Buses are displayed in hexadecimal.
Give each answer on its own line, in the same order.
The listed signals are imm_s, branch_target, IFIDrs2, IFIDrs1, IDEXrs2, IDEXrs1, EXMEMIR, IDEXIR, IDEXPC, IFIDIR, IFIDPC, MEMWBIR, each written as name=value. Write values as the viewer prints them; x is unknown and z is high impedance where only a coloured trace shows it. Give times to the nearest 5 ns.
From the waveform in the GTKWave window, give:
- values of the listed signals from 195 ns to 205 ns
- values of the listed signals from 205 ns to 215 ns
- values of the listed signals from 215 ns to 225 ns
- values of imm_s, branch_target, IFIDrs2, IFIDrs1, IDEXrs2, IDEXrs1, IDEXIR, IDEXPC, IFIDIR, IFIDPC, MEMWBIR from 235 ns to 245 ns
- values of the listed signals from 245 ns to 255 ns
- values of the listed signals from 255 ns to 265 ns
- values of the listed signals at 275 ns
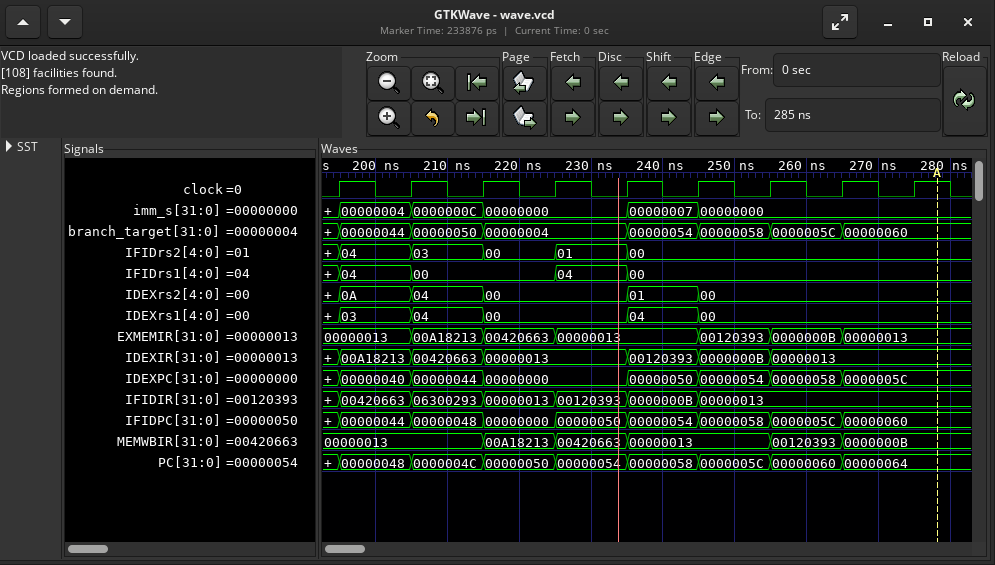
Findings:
imm_s=00000004, branch_target=00000044, IFIDrs2=04, IFIDrs1=04, IDEXrs2=0A, IDEXrs1=03, EXMEMIR=00000013, IDEXIR=00A18213, IDEXPC=00000040, IFIDIR=00420663, IFIDPC=00000044, MEMWBIR=00000013
imm_s=0000000C, branch_target=00000050, IFIDrs2=03, IFIDrs1=00, IDEXrs2=04, IDEXrs1=04, EXMEMIR=00A18213, IDEXIR=00420663, IDEXPC=00000044, IFIDIR=06300293, IFIDPC=00000048, MEMWBIR=00000013
imm_s=00000000, branch_target=00000004, IFIDrs2=00, IFIDrs1=00, IDEXrs2=00, IDEXrs1=00, EXMEMIR=00420663, IDEXIR=00000013, IDEXPC=00000000, IFIDIR=00000013, IFIDPC=00000000, MEMWBIR=00A18213
imm_s=00000007, branch_target=00000054, IFIDrs2=00, IFIDrs1=00, IDEXrs2=01, IDEXrs1=04, IDEXIR=00120393, IDEXPC=00000050, IFIDIR=0000000B, IFIDPC=00000054, MEMWBIR=00000013
imm_s=00000000, branch_target=00000058, IFIDrs2=00, IFIDrs1=00, IDEXrs2=00, IDEXrs1=00, EXMEMIR=00120393, IDEXIR=0000000B, IDEXPC=00000054, IFIDIR=00000013, IFIDPC=00000058, MEMWBIR=00000013
imm_s=00000000, branch_target=0000005C, IFIDrs2=00, IFIDrs1=00, IDEXrs2=00, IDEXrs1=00, EXMEMIR=0000000B, IDEXIR=00000013, IDEXPC=00000058, IFIDIR=00000013, IFIDPC=0000005C, MEMWBIR=00120393
imm_s=00000000, branch_target=00000060, IFIDrs2=00, IFIDrs1=00, IDEXrs2=00, IDEXrs1=00, EXMEMIR=00000013, IDEXIR=00000013, IDEXPC=0000005C, IFIDIR=00000013, IFIDPC=00000060, MEMWBIR=0000000B
